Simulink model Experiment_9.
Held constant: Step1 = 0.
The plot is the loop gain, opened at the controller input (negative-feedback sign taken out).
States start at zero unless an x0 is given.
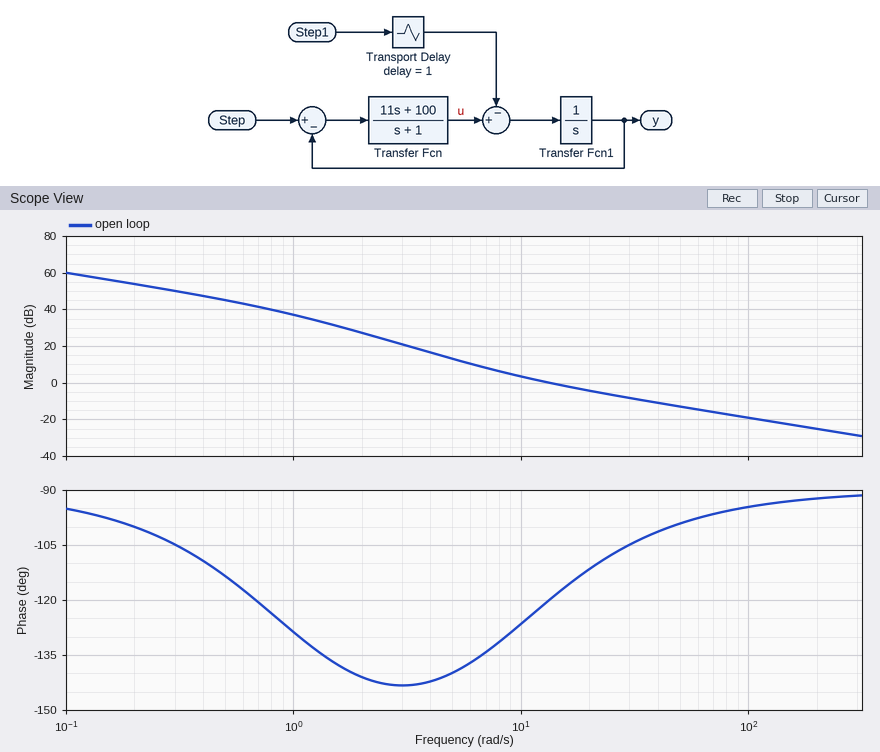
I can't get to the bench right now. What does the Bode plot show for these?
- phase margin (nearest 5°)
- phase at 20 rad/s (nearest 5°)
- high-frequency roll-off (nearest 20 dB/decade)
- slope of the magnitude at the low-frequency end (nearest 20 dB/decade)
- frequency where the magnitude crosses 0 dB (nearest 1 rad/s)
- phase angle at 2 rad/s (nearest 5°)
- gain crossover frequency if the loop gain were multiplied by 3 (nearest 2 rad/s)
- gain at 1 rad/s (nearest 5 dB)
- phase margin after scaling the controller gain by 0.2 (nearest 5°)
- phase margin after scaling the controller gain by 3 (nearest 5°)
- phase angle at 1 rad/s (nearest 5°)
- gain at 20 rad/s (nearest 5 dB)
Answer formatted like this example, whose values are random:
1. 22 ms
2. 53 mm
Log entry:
1. 60°
2. -110°
3. -20 dB/decade
4. -20 dB/decade
5. 13 rad/s
6. -140°
7. 34 rad/s
8. 35 dB
9. 40°
10. 75°
11. -130°
12. -5 dB
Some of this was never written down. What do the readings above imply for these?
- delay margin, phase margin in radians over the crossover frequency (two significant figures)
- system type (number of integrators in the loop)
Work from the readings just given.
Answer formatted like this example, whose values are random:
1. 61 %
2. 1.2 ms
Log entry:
1. 0.081 s
2. 1
